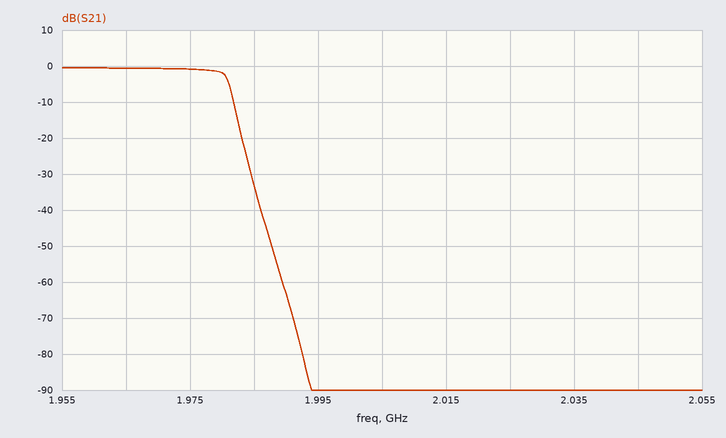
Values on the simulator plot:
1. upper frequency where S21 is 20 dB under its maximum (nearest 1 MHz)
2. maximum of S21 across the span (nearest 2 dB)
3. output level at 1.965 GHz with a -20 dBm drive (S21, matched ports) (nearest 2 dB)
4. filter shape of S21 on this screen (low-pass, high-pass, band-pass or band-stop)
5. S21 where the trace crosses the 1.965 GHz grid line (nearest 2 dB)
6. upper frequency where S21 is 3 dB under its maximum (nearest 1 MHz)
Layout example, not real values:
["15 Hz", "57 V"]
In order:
["1.983 GHz", "0 dB", "-20 dBm", "low-pass", "0 dB", "1.981 GHz"]
